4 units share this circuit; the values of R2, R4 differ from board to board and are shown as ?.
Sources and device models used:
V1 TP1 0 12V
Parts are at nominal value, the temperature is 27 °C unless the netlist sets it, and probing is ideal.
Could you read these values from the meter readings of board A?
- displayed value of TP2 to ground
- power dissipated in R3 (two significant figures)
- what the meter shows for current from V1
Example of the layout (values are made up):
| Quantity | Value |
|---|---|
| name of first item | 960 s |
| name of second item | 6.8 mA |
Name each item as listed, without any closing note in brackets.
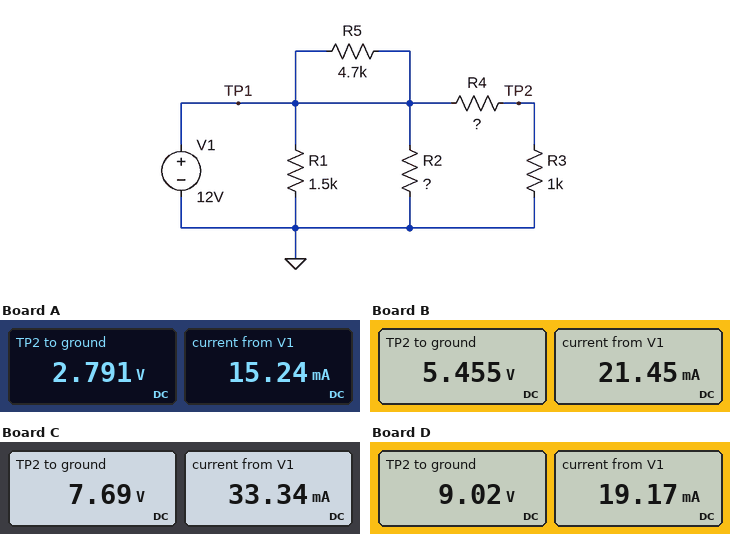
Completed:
| Quantity | Value |
|---|---|
| displayed value of TP2 to ground | 2.791 V |
| power dissipated in R3 | 7.8 mW |
| what the meter shows for current from V1 | 15.24 mA |
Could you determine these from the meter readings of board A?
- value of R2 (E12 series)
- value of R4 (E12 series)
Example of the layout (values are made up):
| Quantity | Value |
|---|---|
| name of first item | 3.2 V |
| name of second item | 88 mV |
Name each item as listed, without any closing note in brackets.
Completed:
| Quantity | Value |
|---|---|
| value of R2 | 2.7 kΩ |
| value of R4 | 3.3 kΩ |
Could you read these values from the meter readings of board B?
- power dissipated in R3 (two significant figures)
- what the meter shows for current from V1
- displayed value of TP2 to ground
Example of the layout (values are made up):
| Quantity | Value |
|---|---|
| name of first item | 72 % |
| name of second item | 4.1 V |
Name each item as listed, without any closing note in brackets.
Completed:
| Quantity | Value |
|---|---|
| power dissipated in R3 | 30 mW |
| what the meter shows for current from V1 | 21.45 mA |
| displayed value of TP2 to ground | 5.455 V |
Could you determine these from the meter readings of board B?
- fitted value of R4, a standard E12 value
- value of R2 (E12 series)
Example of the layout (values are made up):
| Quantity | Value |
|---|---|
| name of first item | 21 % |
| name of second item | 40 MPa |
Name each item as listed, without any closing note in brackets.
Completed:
| Quantity | Value |
|---|---|
| fitted value of R4, a standard E12 value | 1.2 kΩ |
| value of R2 | 1.5 kΩ |
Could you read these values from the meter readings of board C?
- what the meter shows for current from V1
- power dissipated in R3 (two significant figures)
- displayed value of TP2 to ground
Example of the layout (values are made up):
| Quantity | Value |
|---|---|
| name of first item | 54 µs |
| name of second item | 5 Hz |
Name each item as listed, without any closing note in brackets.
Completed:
| Quantity | Value |
|---|---|
| what the meter shows for current from V1 | 33.34 mA |
| power dissipated in R3 | 59 mW |
| displayed value of TP2 to ground | 7.69 V |
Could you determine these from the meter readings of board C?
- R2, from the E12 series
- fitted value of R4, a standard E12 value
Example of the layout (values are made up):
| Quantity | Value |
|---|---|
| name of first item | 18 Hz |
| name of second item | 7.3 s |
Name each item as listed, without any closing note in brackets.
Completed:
| Quantity | Value |
|---|---|
| R2, from the E12 series | 680 Ω |
| fitted value of R4, a standard E12 value | 560 Ω |
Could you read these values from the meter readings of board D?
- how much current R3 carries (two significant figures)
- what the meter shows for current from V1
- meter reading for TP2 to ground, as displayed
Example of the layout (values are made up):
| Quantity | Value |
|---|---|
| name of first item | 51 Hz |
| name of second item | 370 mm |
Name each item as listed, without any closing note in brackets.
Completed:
| Quantity | Value |
|---|---|
| how much current R3 carries | 9.0 mA |
| what the meter shows for current from V1 | 19.17 mA |
| meter reading for TP2 to ground, as displayed | 9.02 V |
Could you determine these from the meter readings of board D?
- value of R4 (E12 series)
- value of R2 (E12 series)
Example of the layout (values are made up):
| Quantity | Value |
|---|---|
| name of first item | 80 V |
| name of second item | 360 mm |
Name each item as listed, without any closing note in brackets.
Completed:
| Quantity | Value |
|---|---|
| value of R4 | 330 Ω |
| value of R2 | 5.6 kΩ |
